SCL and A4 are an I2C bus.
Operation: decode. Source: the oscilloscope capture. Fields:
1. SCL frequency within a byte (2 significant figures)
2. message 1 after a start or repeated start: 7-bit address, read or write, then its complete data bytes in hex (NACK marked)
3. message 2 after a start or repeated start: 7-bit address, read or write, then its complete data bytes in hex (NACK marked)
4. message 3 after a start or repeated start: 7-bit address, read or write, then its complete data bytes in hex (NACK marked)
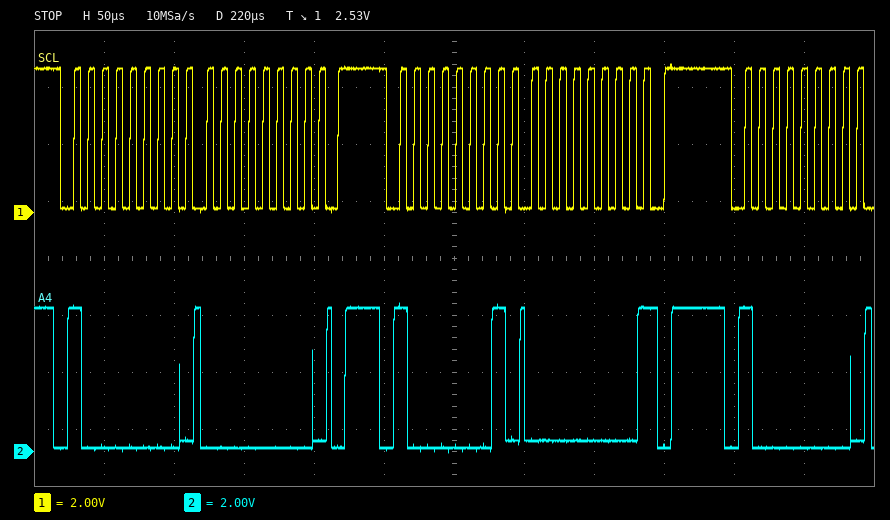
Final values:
100 kHz
0x40 write: 00
0x40 read: 00 NACK
0x40 write
